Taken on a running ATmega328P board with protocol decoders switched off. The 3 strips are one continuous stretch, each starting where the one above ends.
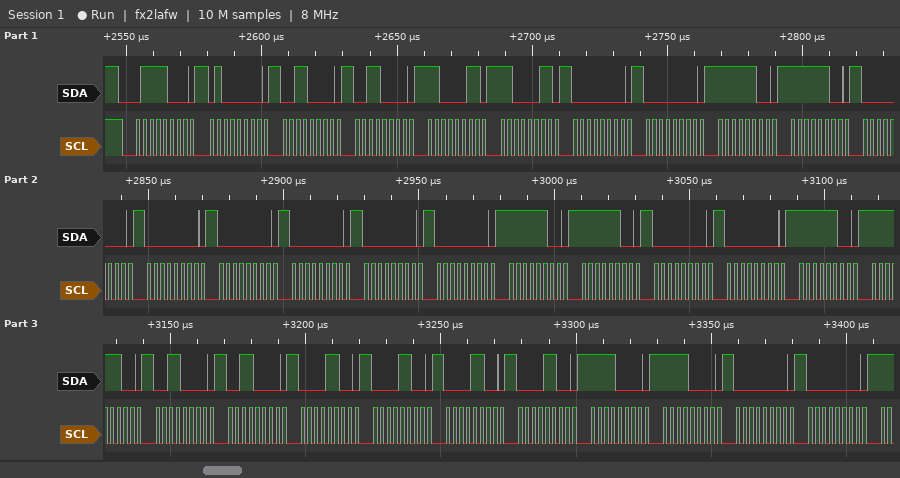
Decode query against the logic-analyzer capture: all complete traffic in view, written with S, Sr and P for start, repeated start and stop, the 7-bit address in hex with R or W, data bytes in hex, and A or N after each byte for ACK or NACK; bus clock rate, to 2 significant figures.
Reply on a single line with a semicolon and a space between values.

S 3CW A 40 A 30 A 30 A C3 A C3 A 00 A 00 A FC A FC A 00 A 00 A 00 A 00 A 00 A 00 A FC A FC A 00 A 00 A FC A FC A 30 A 30 A 0C A 0C A 0C A 0C A F0 A F0 A 00 A 00 A; 400 kHz
